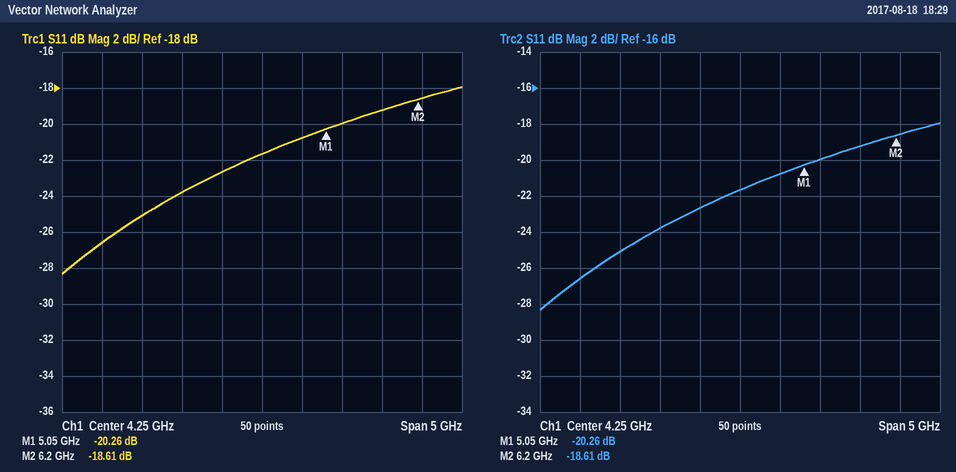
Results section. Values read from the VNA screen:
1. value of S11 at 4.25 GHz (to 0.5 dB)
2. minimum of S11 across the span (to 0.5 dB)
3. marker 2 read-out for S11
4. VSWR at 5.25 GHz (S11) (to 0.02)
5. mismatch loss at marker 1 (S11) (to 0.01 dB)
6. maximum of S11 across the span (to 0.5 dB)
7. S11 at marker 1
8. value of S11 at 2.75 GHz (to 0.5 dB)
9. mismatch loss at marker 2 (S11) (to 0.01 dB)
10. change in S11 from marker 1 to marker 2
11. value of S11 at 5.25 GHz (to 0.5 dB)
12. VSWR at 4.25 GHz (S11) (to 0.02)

-21.5 dB
-28.5 dB
-18.61 dB
1.22
0.04 dB
-18.0 dB
-20.26 dB
-25.0 dB
0.06 dB
1.65 dB
-20.0 dB
1.18
